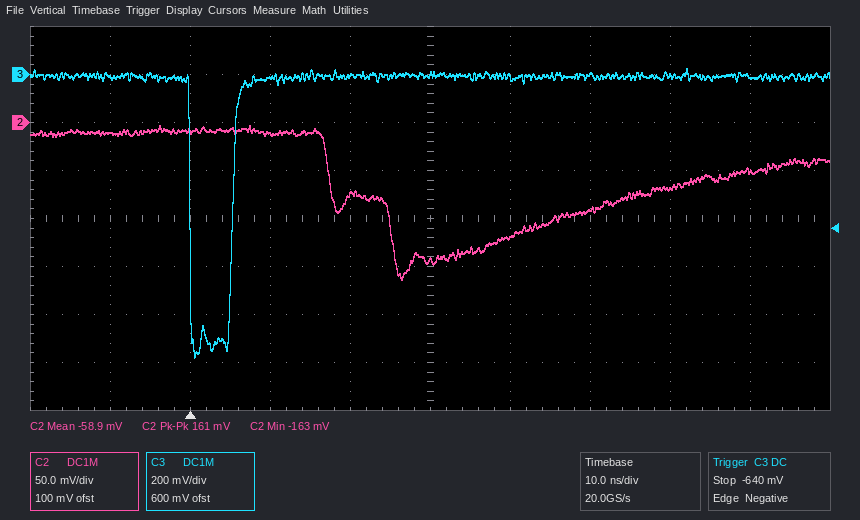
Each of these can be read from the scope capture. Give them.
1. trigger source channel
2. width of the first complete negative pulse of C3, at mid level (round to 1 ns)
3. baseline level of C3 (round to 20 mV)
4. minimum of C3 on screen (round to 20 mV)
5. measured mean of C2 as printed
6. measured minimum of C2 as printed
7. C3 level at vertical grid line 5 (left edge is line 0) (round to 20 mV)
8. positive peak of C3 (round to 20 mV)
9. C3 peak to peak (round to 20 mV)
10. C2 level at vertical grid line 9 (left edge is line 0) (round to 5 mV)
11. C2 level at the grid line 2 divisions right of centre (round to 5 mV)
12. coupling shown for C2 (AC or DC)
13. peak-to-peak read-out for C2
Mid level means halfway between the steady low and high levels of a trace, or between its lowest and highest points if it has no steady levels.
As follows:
C3
5 ns
0 mV
-1.18 V
-58.9 mV
-163 mV
0 mV
20 mV
1.20 V
-50 mV
-90 mV
DC
161 mV
